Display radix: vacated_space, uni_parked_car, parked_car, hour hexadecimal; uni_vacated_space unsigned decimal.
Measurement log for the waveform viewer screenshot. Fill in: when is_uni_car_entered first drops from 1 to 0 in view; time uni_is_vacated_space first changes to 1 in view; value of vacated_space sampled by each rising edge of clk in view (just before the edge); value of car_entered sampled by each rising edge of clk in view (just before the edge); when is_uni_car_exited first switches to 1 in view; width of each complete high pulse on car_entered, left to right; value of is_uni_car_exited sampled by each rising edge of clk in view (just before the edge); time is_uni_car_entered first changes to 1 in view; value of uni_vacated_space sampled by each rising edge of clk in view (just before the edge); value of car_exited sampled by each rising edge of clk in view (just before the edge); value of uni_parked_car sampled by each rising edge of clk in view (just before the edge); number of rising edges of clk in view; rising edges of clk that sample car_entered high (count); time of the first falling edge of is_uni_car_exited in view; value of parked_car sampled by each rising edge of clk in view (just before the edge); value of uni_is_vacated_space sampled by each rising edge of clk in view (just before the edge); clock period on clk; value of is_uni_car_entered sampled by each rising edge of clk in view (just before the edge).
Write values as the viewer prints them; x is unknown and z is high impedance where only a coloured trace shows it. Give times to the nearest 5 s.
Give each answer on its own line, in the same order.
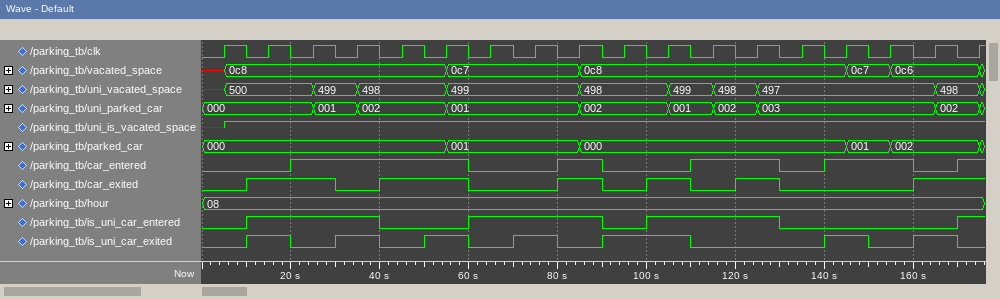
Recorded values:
40 s
5 s
x, 0c8, 0c8, 0c8, 0c8, 0c8, 0c7, 0c7, 0c7, 0c8, 0c8, 0c8, 0c8, 0c8, 0c8, 0c7, 0c6, 0c6
0 0 1 1 1 1 0 0 1 0 0 1 1 0 1 1 0 1
10 s
40 s, 10 s, 20 s, 20 s
0 1 0 1 0 1 0 1 0 1 1 0 0 0 1 0 1 0
10 s
x, 500, 500, 499, 498, 498, 499, 499, 499, 498, 498, 499, 498, 497, 497, 497, 497, 498
0 1 1 0 1 1 0 0 1 0 1 0 1 0 0 0 1 1
000, 000, 000, 001, 002, 002, 001, 001, 001, 002, 002, 001, 002, 003, 003, 003, 003, 002
18
10
20 s
000, 000, 000, 000, 000, 000, 001, 001, 001, 000, 000, 000, 000, 000, 000, 001, 002, 002
x 1 1 1 1 1 1 1 1 1 1 1 1 1 1 1 1 1
10 s
0 1 1 1 0 0 1 1 1 0 1 1 1 0 0 0 0 1
